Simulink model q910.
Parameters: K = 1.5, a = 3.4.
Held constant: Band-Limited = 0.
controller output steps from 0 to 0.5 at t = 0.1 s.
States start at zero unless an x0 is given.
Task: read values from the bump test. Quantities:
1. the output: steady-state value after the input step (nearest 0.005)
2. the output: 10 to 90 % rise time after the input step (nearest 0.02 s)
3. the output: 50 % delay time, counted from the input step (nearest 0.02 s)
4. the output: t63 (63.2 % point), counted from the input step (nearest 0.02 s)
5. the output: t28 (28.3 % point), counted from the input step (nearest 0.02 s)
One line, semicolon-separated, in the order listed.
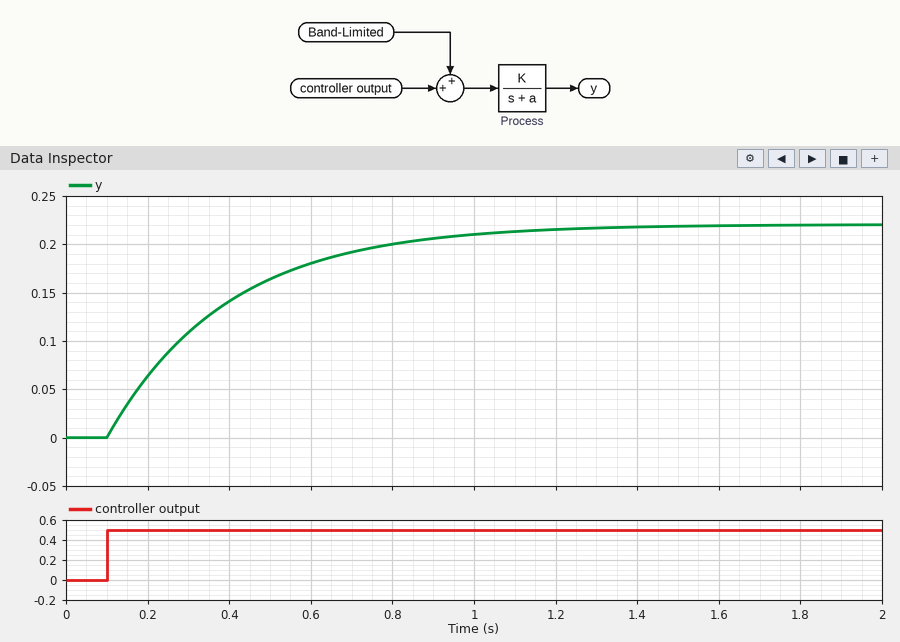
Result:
0.220; 0.64 s; 0.20 s; 0.30 s; 0.10 s
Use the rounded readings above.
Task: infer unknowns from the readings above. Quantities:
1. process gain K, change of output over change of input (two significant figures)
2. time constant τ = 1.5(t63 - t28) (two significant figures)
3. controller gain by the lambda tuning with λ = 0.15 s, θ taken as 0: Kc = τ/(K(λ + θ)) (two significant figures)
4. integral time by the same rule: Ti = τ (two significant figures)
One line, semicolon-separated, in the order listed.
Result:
0.44; 0.30 s; 4.5; 0.30 s
